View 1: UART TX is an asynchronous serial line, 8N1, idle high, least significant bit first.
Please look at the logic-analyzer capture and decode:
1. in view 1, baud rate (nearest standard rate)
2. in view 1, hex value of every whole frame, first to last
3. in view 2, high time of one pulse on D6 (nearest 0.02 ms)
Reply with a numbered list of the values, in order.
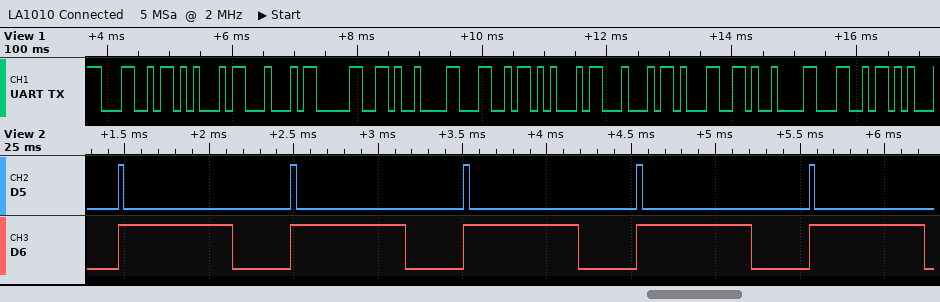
1. 9600 baud
2. 4C 45 44 30 09 4C 45 44 31 09 4C
3. 0.68 ms
